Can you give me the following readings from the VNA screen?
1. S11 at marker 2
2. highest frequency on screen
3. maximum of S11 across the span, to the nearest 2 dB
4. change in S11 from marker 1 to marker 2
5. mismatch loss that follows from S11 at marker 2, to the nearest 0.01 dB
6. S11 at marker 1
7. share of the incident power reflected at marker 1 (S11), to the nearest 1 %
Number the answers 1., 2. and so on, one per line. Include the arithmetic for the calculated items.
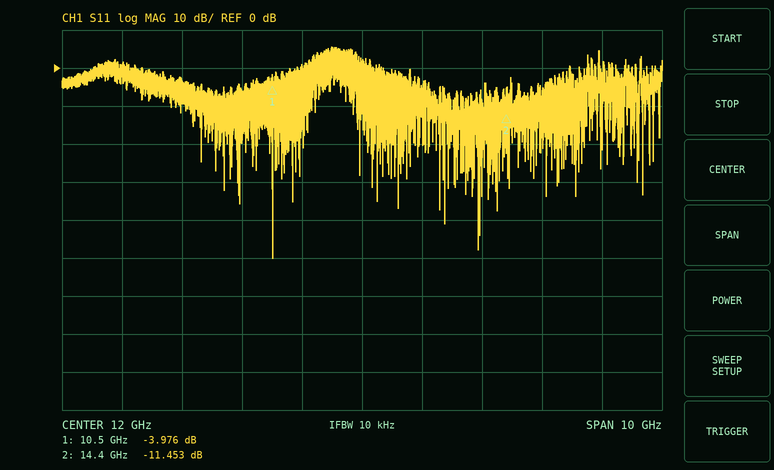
1. -11.453 dB
2. 17 GHz
3. 6 dB
4. -11.453 − (-3.976) = -7.477 dB
5. −10 log10(1 − 10^(-11.453/10)) ≈ 0.32 dB
6. -3.976 dB
7. 10^(-3.976/10) ≈ 40 %
